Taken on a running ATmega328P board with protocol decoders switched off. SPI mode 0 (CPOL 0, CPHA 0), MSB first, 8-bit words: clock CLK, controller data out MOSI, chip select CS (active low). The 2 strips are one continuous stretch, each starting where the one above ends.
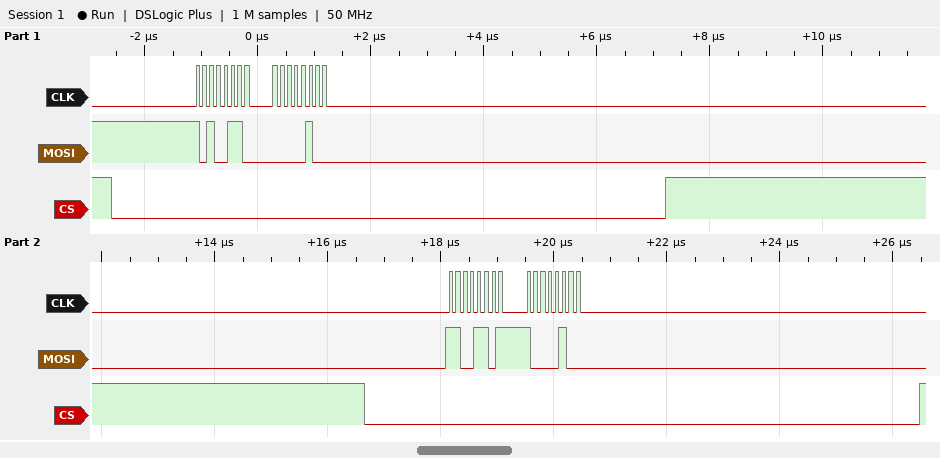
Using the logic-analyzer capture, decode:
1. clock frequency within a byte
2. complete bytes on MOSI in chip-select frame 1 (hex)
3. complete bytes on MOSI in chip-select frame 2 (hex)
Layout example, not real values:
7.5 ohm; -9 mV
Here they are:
8 MHz; A6 04; CD 84
